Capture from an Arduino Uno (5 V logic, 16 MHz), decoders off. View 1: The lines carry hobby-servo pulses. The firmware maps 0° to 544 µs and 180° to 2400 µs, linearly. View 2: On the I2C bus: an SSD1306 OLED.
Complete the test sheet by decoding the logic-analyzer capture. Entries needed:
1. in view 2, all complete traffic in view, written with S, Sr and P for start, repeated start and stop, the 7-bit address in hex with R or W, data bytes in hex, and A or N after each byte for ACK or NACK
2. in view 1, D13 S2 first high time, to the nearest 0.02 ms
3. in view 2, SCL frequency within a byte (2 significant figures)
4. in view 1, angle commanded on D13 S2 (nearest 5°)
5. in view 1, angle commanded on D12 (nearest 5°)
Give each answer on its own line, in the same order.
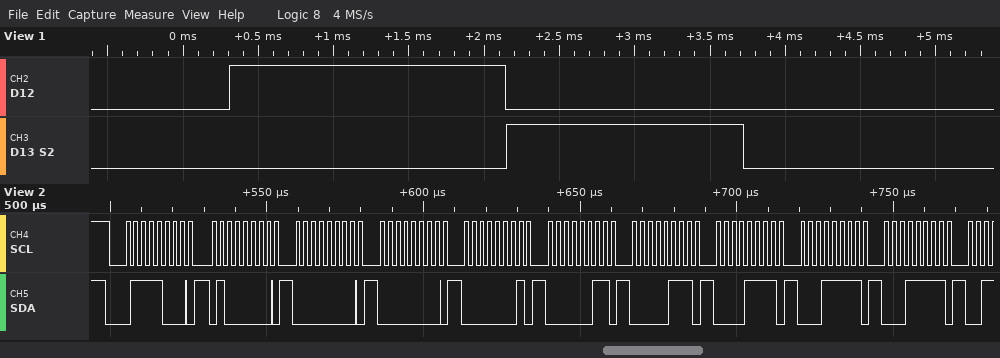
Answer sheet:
S 3CW A 40 A 00 A 00 A 01 A 03 A 07 A 0F A 1F A 1F A
1.58 ms
400 kHz
100°
125°
